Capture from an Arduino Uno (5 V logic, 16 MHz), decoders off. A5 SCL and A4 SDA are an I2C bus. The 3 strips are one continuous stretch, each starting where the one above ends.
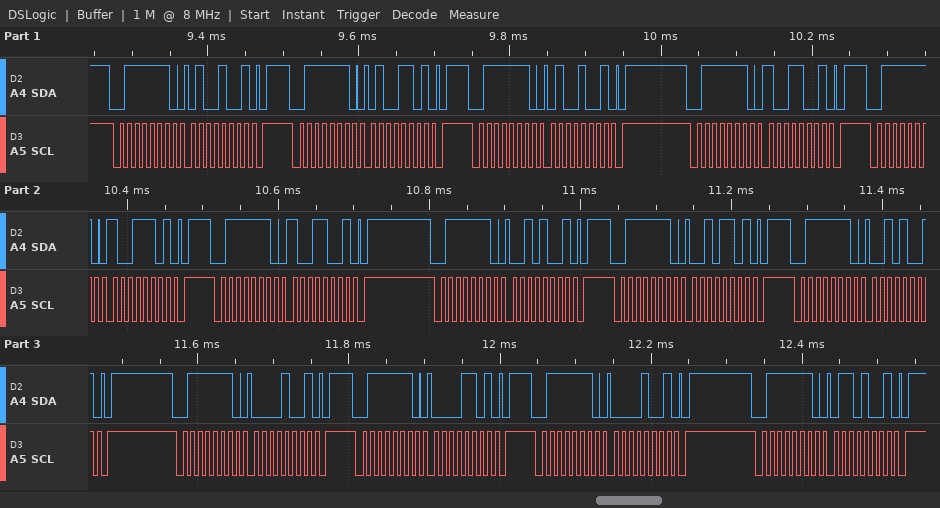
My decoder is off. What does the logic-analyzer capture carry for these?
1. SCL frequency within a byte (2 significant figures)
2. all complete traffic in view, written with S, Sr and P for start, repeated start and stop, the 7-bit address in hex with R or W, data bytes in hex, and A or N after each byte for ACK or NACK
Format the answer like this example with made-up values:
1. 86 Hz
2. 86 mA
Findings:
1. 100 kHz
2. S 3FW A 49 A P S 3FW A 4D A P S 3FW A 49 A P S 3FW A 99 A P S 3FW A 9D A P S 3FW A 99 A P S 3FW A 29 A P S 3FW A 2D A P S 3FW A 29 A P S 3FW A 09 A P S 3FW A 0D A P S 3FW A 09 A P S 3FW A 69 A P
